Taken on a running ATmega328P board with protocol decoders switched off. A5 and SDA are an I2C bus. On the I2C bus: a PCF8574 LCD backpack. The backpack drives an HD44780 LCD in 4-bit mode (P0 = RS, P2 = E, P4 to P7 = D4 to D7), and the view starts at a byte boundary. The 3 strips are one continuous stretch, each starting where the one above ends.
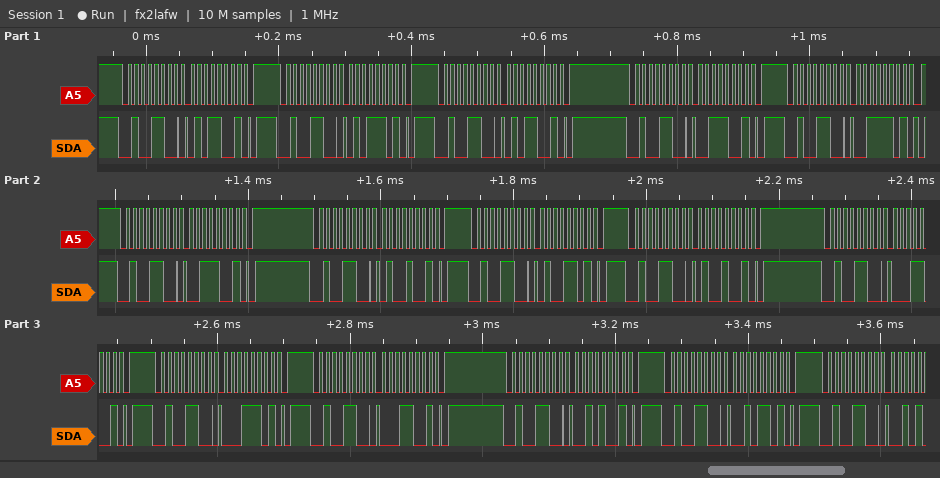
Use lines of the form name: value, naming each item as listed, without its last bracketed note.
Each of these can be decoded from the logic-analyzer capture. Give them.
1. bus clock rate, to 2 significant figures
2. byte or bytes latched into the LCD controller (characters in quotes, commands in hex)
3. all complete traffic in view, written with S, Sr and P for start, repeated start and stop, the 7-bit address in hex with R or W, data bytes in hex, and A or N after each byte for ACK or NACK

bus clock rate, to 2 significant figures: 100 kHz
byte or bytes latched into the LCD controller: 'S' 'A'
all complete traffic in view, written with S, Sr and P for start, repeated start and stop, the 7-bit address in hex with R or W, data bytes in hex, and A or N after each byte for ACK or NACK: S 26W A 59 A P S 26W A 5D A P S 26W A 59 A P S 26W A 39 A P S 26W A 3D A P S 26W A 39 A P S 26W A 49 A P S 26W A 4D A P S 26W A 49 A P S 26W A 19 A P S 26W A 1D A P S 26W A 19 A P S 26W A 29 A P S 26W A 2D A P S 26W A
